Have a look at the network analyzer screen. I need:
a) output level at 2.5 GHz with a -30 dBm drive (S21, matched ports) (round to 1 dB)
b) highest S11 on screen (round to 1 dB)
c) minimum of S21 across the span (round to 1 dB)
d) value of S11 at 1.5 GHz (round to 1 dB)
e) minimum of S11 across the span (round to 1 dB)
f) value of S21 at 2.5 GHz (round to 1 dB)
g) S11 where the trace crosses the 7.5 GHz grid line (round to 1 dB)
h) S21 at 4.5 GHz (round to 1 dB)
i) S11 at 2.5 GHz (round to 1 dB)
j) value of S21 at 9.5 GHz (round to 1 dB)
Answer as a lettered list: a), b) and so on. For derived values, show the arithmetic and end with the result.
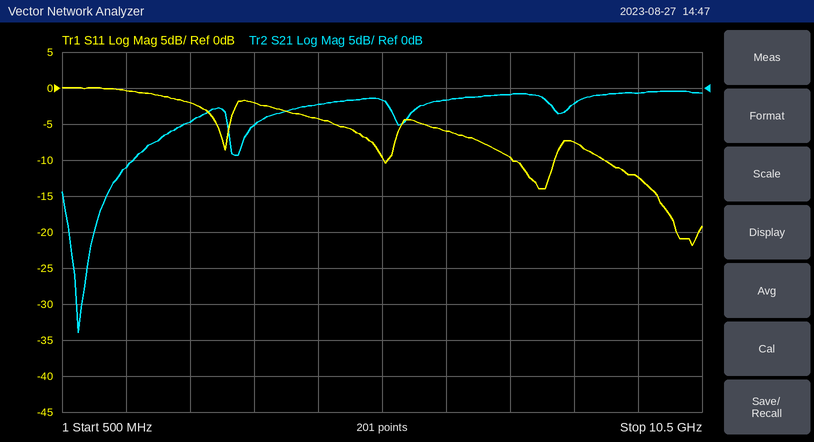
a) -30 dBm + (-5 dB) = -35 dBm
b) 0 dB
c) -34 dB
d) 0 dB
e) -22 dB
f) -5 dB
g) -10 dB
h) -2 dB
i) -2 dB
j) -1 dB
